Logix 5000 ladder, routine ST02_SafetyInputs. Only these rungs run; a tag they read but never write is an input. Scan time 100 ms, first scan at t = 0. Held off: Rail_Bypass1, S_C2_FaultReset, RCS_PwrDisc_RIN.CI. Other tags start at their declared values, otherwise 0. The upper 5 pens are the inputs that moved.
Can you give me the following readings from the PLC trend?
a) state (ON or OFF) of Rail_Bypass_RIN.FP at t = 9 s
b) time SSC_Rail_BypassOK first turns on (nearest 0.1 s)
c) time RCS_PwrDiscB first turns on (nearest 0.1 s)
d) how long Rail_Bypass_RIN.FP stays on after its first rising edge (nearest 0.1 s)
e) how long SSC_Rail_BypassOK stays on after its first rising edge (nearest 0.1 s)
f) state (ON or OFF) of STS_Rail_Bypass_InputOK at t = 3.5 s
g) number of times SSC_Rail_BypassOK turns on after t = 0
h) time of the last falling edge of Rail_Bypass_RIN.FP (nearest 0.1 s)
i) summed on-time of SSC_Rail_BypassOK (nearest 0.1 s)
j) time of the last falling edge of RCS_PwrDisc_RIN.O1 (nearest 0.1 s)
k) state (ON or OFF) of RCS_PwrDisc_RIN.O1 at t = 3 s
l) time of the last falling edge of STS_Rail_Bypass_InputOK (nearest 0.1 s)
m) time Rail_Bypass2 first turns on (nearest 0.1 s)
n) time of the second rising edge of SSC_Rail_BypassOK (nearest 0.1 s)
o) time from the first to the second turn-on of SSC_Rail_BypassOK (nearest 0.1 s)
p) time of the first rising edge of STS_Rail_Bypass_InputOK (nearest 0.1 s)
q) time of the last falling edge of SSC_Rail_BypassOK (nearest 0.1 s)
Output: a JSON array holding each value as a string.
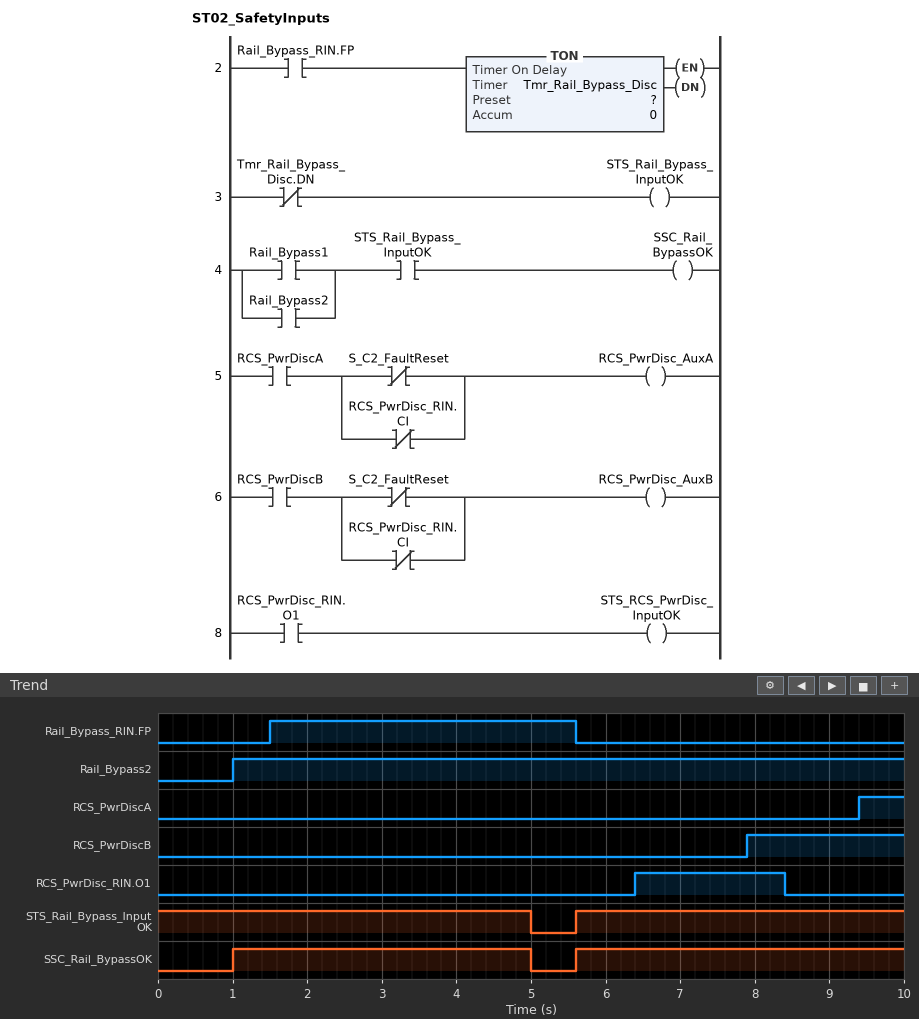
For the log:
["OFF", "1.0 s", "7.9 s", "4.1 s", "4.0 s", "ON", "2", "5.6 s", "8.4 s", "8.4 s", "OFF", "5.0 s", "1.0 s", "5.6 s", "4.6 s", "5.6 s", "5.0 s"]
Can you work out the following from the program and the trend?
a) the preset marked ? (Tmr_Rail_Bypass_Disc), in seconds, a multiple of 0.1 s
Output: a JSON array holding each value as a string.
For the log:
["3.5 s"]
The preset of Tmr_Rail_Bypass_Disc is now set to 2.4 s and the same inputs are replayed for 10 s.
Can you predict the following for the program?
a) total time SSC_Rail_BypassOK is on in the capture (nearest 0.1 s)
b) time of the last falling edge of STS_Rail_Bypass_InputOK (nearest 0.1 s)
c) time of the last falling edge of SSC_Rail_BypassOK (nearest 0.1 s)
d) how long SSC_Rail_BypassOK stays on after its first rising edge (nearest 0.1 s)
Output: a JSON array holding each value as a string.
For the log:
["7.3 s", "3.9 s", "3.9 s", "2.9 s"]
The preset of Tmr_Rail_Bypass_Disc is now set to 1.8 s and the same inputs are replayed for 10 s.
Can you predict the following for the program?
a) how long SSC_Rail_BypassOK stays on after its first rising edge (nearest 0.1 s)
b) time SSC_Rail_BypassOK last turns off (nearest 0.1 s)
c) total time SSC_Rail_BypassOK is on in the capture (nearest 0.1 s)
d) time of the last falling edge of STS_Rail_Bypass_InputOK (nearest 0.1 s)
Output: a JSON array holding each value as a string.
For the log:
["2.3 s", "3.3 s", "6.7 s", "3.3 s"]
